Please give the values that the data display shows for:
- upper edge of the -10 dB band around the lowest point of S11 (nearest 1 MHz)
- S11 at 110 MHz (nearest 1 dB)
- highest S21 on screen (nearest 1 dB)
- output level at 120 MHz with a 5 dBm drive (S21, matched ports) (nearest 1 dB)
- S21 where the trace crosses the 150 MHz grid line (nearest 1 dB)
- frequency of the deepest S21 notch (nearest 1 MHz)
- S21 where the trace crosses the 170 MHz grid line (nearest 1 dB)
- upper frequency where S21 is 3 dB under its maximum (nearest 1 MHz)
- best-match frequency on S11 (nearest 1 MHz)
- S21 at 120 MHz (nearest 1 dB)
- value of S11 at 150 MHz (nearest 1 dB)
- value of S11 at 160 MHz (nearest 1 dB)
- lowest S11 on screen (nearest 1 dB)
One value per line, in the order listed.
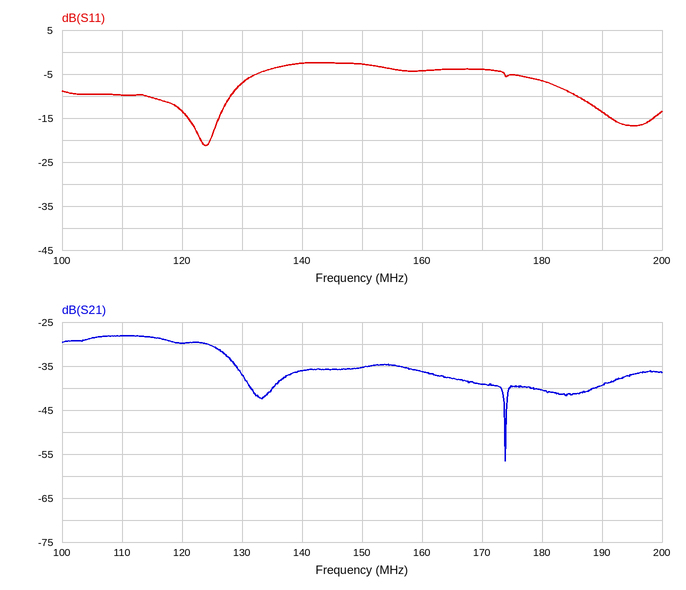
128 MHz
-10 dB
-28 dB
-25 dBm
-35 dB
174 MHz
-39 dB
126 MHz
124 MHz
-30 dB
-3 dB
-4 dB
-21 dB
